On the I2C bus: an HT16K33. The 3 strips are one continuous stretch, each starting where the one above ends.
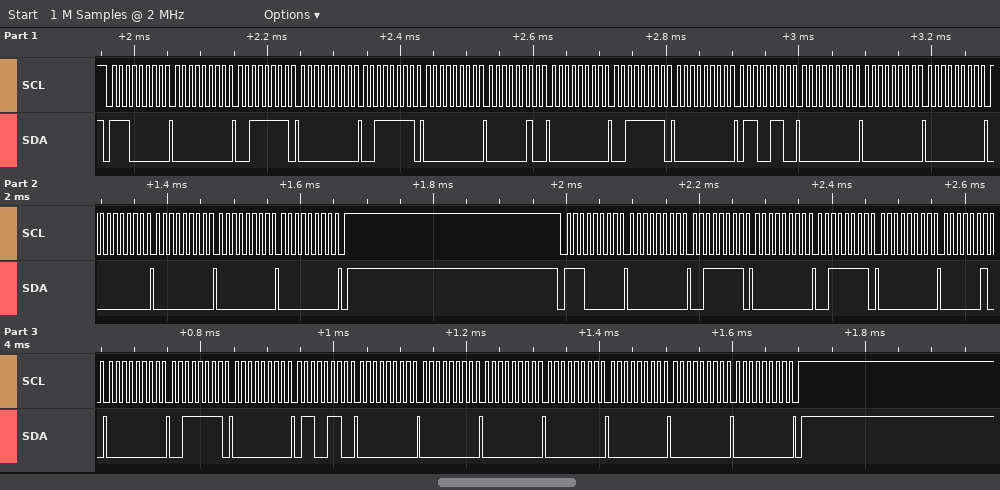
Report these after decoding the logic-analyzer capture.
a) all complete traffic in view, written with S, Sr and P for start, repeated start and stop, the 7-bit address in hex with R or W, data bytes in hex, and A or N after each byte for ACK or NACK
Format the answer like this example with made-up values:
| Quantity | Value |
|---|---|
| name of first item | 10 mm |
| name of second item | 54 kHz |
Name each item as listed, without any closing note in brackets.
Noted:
| Quantity | Value |
|---|---|
| all complete traffic in view, written with S, Sr and P for start, repeated start and stop, the 7-bit address in hex with R or W, data bytes in hex, and A or N after each byte for ACK or NACK | S 70W A 00 A 3F A 00 A 3F A 00 A 02 A 00 A 3F A 00 A 66 A 00 A 00 A 00 A 00 A 00 A 00 A 00 A P S 70W A 00 A 3F A 00 A 3F A 00 A 02 A 00 A 3F A 00 A 66 A 00 A 00 A 00 A 00 A 00 A 00 A 00 A P |
